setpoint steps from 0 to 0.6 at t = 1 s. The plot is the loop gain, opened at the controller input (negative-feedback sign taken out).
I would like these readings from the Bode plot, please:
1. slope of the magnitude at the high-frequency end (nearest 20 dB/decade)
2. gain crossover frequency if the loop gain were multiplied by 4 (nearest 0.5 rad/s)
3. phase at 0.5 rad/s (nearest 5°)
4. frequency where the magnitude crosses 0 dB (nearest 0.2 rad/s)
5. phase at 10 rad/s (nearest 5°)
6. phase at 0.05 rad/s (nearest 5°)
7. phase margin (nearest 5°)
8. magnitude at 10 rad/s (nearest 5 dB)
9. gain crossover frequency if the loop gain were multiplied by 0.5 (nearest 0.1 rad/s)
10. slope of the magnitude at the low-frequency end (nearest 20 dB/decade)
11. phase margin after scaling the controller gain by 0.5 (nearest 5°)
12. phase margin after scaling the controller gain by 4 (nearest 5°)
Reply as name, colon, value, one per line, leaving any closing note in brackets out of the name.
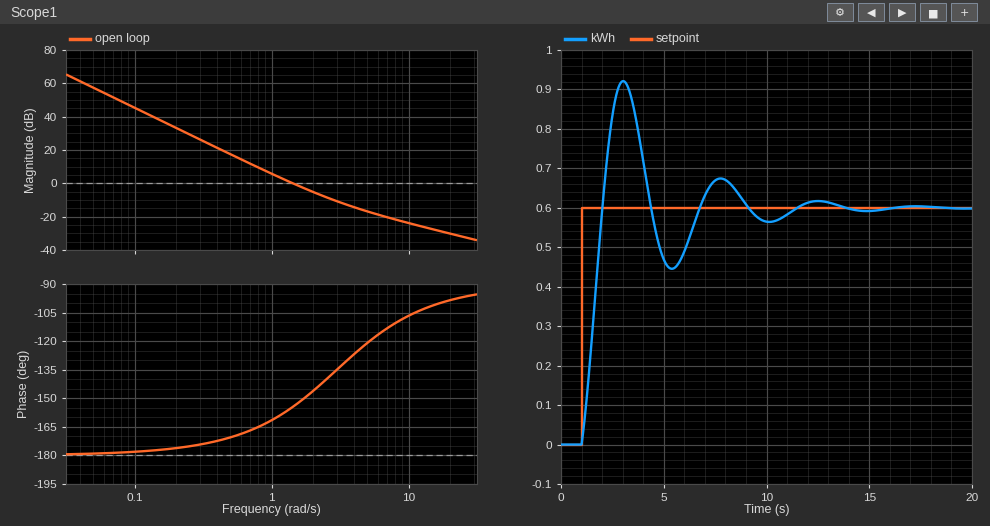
slope of the magnitude at the high-frequency end: -20 dB/decade
gain crossover frequency if the loop gain were multiplied by 4: 3.5 rad/s
phase at 0.5 rad/s: -170°
frequency where the magnitude crosses 0 dB: 1.4 rad/s
phase at 10 rad/s: -105°
phase at 0.05 rad/s: -180°
phase margin: 25°
magnitude at 10 rad/s: -25 dB
gain crossover frequency if the loop gain were multiplied by 0.5: 1.0 rad/s
slope of the magnitude at the low-frequency end: -40 dB/decade
phase margin after scaling the controller gain by 0.5: 20°
phase margin after scaling the controller gain by 4: 50°
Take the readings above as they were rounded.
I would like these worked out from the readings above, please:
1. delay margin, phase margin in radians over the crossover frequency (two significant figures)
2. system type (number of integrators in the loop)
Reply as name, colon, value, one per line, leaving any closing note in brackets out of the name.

delay margin, phase margin in radians over the crossover frequency: 0.31 s
system type: 2
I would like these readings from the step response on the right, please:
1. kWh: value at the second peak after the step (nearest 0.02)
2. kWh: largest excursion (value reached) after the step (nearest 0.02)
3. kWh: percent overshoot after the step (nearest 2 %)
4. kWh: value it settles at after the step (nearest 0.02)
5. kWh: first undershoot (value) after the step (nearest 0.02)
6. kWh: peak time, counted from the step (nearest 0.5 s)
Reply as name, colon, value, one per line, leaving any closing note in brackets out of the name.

kWh: value at the second peak after the step: 0.68
kWh: largest excursion (value reached) after the step: 0.92
kWh: percent overshoot after the step: 54 %
kWh: value it settles at after the step: 0.60
kWh: first undershoot (value) after the step: 0.44
kWh: peak time, counted from the step: 2.0 s
